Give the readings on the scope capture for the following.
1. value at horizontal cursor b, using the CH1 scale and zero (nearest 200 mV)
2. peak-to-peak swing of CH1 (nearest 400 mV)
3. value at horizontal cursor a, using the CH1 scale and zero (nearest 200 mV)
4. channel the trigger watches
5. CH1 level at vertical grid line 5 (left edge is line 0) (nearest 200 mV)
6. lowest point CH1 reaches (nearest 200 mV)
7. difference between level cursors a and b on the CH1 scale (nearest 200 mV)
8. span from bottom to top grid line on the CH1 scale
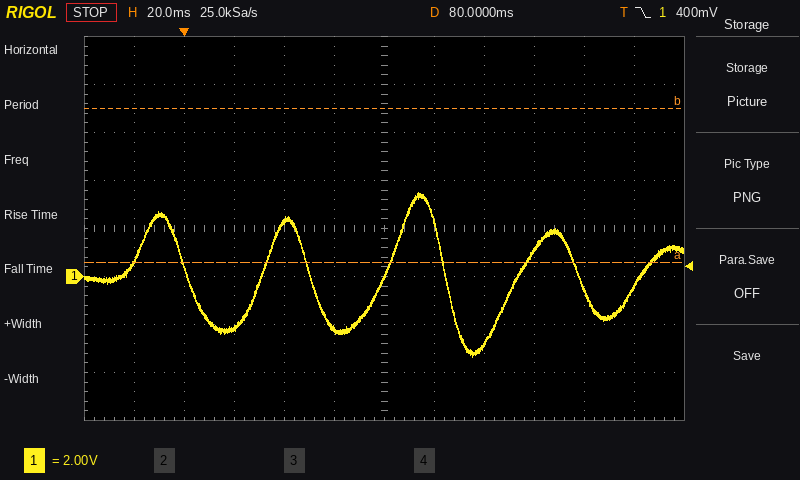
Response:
7.0 V
6.8 V
600 mV
CH1
-2.2 V
-3.4 V
6.4 V
16 V
